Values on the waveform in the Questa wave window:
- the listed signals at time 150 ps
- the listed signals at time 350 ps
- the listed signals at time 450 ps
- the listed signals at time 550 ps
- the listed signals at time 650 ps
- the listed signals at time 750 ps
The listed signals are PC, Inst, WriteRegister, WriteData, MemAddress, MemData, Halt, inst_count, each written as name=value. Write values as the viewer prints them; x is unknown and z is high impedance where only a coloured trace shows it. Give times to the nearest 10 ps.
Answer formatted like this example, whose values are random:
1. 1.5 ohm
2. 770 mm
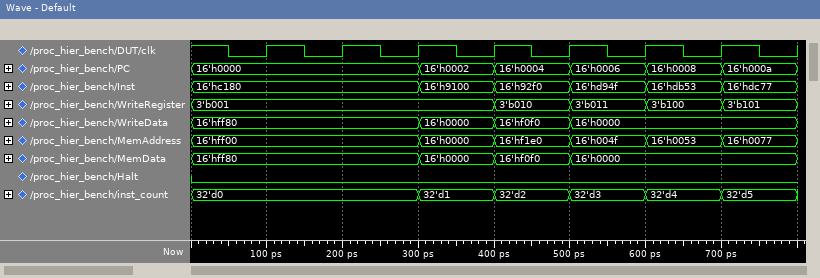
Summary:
1. PC=16'h0000, Inst=16'hc180, WriteRegister=3'b001, WriteData=16'hff80, MemAddress=16'hff00, MemData=16'hff80, Halt=0, inst_count=32'd0
2. PC=16'h0002, Inst=16'h9100, WriteRegister=3'b001, WriteData=16'h0000, MemAddress=16'h0000, MemData=16'h0000, Halt=0, inst_count=32'd1
3. PC=16'h0004, Inst=16'h92f0, WriteRegister=3'b010, WriteData=16'hf0f0, MemAddress=16'hf1e0, MemData=16'hf0f0, Halt=0, inst_count=32'd2
4. PC=16'h0006, Inst=16'hd94f, WriteRegister=3'b011, WriteData=16'h0000, MemAddress=16'h004f, MemData=16'h0000, Halt=0, inst_count=32'd3
5. PC=16'h0008, Inst=16'hdb53, WriteRegister=3'b100, WriteData=16'h0000, MemAddress=16'h0053, MemData=16'h0000, Halt=0, inst_count=32'd4
6. PC=16'h000a, Inst=16'hdc77, WriteRegister=3'b101, WriteData=16'h0000, MemAddress=16'h0077, MemData=16'h0000, Halt=0, inst_count=32'd5
